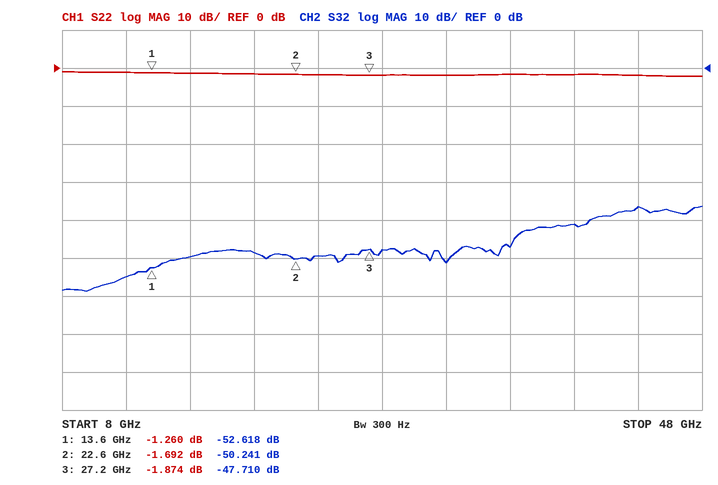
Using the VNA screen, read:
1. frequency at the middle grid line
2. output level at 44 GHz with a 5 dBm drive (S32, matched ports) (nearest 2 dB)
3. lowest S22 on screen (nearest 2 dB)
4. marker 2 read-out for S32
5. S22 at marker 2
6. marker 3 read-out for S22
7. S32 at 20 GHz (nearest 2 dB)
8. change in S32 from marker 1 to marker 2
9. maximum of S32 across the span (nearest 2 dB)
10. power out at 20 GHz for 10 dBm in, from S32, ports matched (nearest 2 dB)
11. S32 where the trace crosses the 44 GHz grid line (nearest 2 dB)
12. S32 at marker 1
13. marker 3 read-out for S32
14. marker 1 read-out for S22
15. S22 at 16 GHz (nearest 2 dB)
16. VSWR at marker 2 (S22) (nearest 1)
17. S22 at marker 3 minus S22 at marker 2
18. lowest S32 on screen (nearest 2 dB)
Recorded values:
28 GHz
-32 dBm
-2 dB
-50.241 dB
-1.692 dB
-1.874 dB
-48 dB
2.377 dB
-36 dB
-38 dBm
-36 dB
-52.618 dB
-47.710 dB
-1.260 dB
-2 dB
10
-0.182 dB
-58 dB
